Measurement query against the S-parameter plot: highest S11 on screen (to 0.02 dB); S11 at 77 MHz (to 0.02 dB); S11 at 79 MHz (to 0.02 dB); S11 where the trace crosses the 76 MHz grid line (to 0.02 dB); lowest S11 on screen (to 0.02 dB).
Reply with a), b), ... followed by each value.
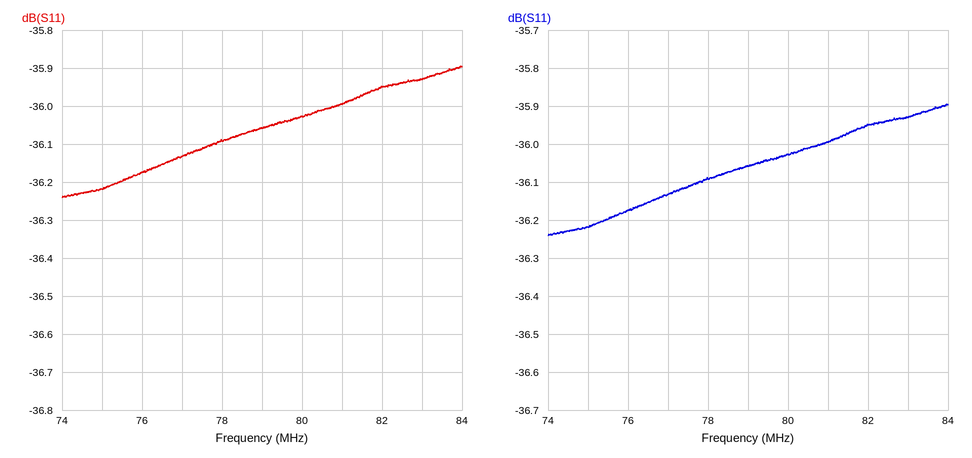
a) -35.90 dB
b) -36.14 dB
c) -36.06 dB
d) -36.18 dB
e) -36.24 dB
